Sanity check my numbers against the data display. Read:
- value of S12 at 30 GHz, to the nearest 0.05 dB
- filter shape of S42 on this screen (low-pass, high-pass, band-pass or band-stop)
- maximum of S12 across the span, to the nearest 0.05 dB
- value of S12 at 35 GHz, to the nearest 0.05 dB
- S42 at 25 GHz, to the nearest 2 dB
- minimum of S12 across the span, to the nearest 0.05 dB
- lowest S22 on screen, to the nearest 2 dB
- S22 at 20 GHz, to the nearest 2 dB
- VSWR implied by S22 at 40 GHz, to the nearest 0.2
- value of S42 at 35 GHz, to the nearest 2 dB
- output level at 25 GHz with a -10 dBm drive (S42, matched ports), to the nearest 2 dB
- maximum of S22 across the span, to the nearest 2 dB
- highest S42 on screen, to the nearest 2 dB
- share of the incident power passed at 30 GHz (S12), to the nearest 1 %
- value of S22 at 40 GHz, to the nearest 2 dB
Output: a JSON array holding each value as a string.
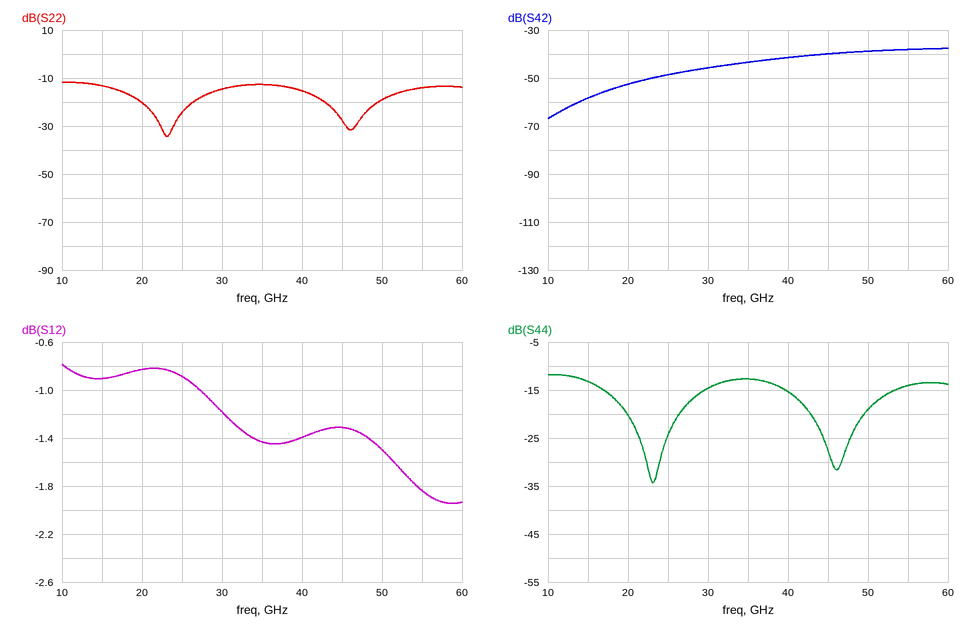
["-1.20 dB", "high-pass", "-0.80 dB", "-1.45 dB", "-48 dB", "-1.95 dB", "-34 dB", "-20 dB", "1.4", "-44 dB", "-58 dBm", "-12 dB", "-38 dB", "76 %", "-16 dB"]
